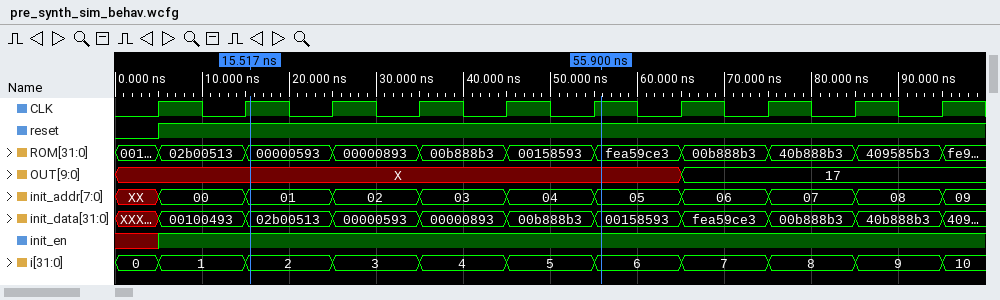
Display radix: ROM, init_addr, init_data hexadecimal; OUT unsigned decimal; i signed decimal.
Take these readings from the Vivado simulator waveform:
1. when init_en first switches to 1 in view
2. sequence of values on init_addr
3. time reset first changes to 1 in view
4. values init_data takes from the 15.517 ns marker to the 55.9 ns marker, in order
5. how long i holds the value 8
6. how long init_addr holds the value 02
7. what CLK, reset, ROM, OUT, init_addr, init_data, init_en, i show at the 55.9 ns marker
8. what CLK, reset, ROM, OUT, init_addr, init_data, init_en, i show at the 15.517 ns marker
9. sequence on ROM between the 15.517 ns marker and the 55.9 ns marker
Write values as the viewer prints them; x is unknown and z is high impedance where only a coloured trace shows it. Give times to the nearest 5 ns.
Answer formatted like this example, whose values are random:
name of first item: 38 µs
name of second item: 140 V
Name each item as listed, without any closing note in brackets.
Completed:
when init_en first switches to 1 in view: 5 ns
sequence of values on init_addr: XX, 00, 01, 02, 03, 04, 05, 06, 07, 08, 09
time reset first changes to 1 in view: 5 ns
values init_data takes from the 15.517 ns marker to the 55.9 ns marker, in order: 02b00513, 00000593, 00000893, 00b888b3, 00158593
how long i holds the value 8: 10 ns
how long init_addr holds the value 02: 10 ns
what CLK, reset, ROM, OUT, init_addr, init_data, init_en, i show at the 55.9 ns marker: CLK=1, reset=1, ROM=fea59ce3, OUT=X, init_addr=05, init_data=00158593, init_en=1, i=6
what CLK, reset, ROM, OUT, init_addr, init_data, init_en, i show at the 15.517 ns marker: CLK=1, reset=1, ROM=00000593, OUT=X, init_addr=01, init_data=02b00513, init_en=1, i=2
sequence on ROM between the 15.517 ns marker and the 55.9 ns marker: 00000593, 00000893, 00b888b3, 00158593, fea59ce3
